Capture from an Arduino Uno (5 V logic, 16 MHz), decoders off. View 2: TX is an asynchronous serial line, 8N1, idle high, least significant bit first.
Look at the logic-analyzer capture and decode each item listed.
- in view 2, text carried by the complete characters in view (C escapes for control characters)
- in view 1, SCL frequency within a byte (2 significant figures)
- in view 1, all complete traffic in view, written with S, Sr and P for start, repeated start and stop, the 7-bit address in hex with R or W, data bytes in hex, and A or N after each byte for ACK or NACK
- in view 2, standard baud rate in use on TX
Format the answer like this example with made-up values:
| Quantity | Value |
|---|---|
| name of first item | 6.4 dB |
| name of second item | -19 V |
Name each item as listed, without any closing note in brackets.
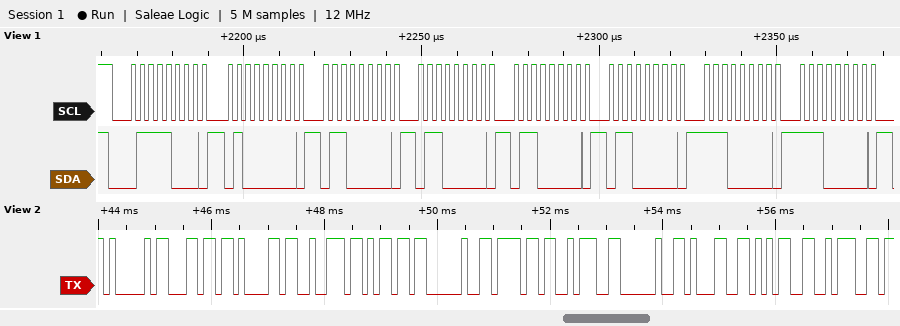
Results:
| Quantity | Value |
|---|---|
| in view 2, text carried by the complete characters in view | "Alarm o: 15:" |
| in view 1, SCL frequency within a byte | 400 kHz |
| in view 1, all complete traffic in view, written with S, Sr and P for start, repeated start and stop, the 7-bit address in hex with R or W, data bytes in hex, and A or N after each byte for ACK or NACK | S 3CW A 40 A 60 A 60 A 60 A 60 A E0 A E0 A |
| in view 2, standard baud rate in use on TX | 9600 baud |
